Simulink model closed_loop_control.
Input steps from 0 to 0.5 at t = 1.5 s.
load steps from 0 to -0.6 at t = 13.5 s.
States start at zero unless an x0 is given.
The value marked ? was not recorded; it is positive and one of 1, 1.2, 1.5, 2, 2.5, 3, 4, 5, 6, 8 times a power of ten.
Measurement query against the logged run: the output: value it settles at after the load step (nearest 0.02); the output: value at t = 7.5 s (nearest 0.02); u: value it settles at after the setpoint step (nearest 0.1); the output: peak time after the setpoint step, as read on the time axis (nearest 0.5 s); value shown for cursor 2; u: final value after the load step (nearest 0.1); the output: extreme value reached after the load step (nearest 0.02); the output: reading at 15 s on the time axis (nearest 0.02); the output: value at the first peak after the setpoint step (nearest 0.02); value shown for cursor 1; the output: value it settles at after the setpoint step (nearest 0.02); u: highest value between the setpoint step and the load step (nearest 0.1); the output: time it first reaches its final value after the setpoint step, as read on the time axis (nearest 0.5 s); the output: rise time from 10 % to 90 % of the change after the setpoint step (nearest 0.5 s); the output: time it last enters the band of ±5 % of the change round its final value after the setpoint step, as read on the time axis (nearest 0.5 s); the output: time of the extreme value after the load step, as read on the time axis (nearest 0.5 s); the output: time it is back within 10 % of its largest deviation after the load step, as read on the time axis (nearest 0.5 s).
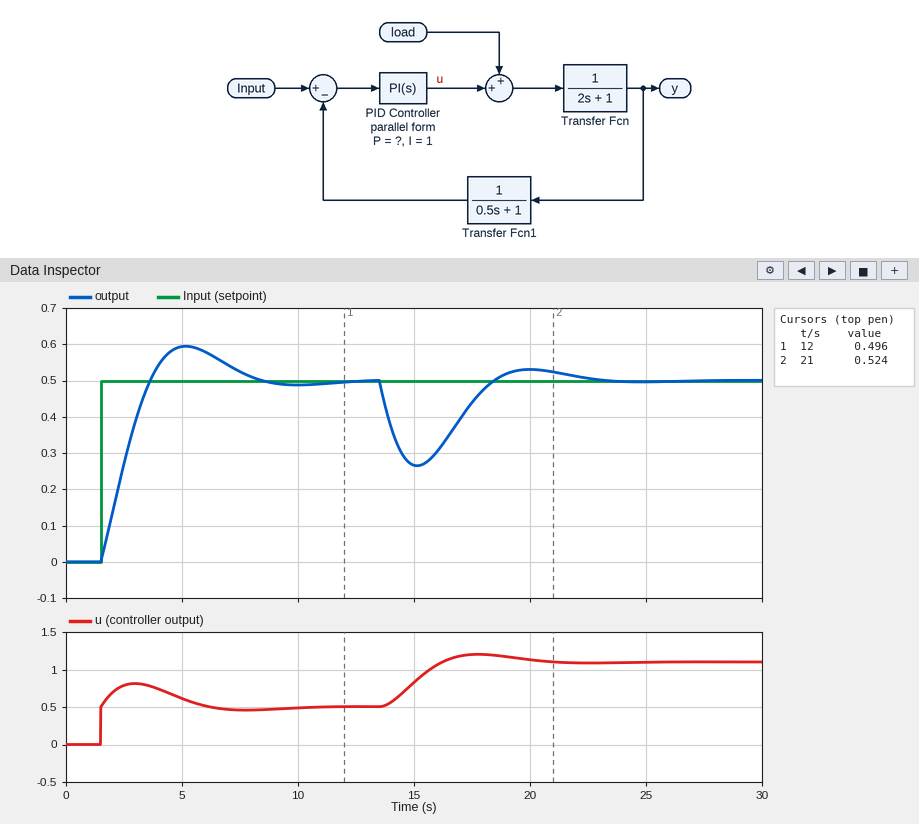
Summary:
0.50
0.52
0.5
5.0 s
0.524
1.1
0.26
0.26
0.60
0.496
0.50
0.8
3.5 s
1.5 s
7.5 s
15.0 s
21.0 s
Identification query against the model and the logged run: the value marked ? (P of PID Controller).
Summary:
1
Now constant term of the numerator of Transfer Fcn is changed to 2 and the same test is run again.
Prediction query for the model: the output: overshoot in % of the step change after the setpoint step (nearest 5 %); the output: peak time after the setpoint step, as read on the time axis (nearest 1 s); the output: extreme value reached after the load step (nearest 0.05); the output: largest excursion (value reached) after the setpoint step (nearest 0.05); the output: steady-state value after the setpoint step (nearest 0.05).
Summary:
35 %
4 s
0.15
0.65
0.50
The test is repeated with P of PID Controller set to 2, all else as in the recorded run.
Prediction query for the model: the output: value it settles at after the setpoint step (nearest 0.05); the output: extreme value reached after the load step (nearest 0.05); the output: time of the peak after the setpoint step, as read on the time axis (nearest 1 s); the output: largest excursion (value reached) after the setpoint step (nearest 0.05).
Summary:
0.50
0.30
4 s
0.55
